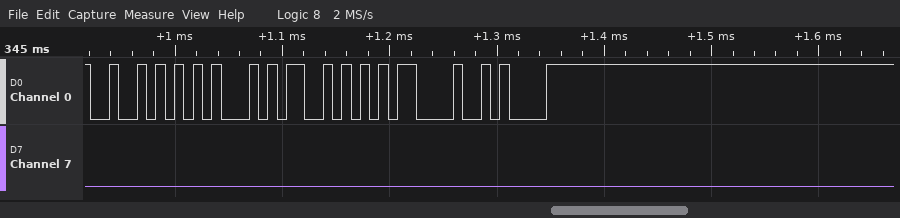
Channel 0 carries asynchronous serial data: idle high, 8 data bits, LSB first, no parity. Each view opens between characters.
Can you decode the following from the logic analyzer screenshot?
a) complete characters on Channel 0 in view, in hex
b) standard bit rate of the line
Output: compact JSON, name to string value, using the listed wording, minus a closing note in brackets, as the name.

{"complete characters on Channel 0 in view, in hex": "52, 45, 53, 0D, 0A", "standard bit rate of the line": "115200 baud"}
